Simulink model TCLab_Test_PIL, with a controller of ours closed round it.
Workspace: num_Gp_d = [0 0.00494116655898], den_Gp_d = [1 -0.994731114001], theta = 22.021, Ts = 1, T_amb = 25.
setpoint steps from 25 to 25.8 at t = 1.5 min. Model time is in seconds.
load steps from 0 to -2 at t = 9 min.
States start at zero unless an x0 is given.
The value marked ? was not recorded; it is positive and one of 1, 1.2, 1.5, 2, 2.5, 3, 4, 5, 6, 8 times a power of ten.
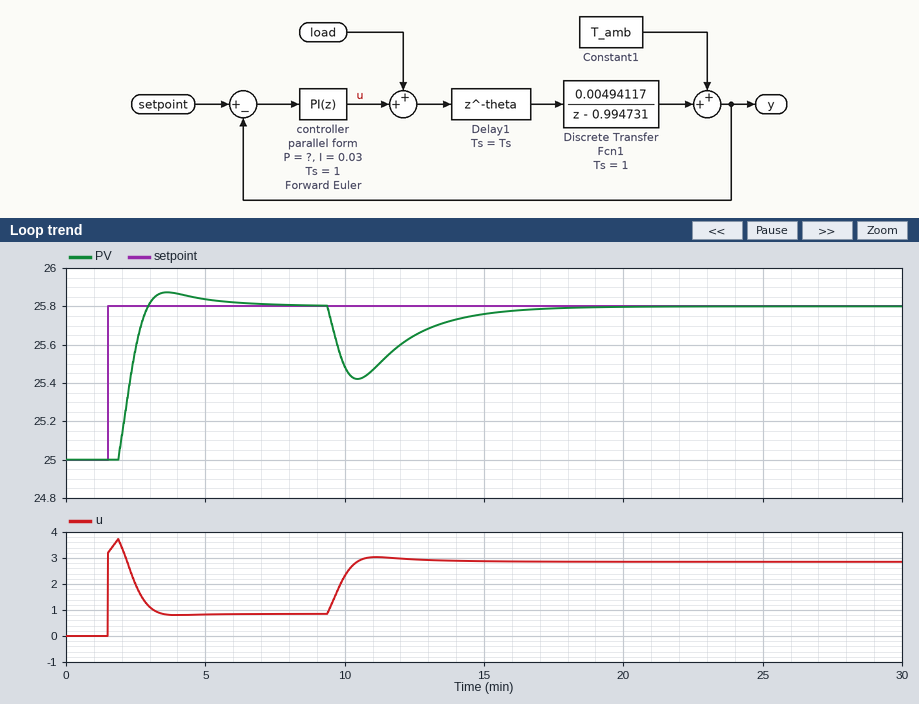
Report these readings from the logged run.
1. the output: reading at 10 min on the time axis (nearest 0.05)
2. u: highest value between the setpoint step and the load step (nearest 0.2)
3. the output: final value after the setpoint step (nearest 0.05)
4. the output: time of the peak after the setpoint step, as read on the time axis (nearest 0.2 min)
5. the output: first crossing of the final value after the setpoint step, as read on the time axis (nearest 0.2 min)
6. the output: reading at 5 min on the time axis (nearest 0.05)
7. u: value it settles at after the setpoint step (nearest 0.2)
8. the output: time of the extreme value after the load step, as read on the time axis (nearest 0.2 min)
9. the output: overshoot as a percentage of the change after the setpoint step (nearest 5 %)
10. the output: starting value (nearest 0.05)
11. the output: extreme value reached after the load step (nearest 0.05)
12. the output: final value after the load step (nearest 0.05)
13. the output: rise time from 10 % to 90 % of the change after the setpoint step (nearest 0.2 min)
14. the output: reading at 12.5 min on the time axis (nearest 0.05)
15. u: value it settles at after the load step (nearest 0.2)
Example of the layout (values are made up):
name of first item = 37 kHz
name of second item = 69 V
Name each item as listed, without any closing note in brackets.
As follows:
the output: reading at 10 min on the time axis = 25.50
u: highest value between the setpoint step and the load step = 3.8
the output: final value after the setpoint step = 25.80
the output: time of the peak after the setpoint step, as read on the time axis = 3.6 min
the output: first crossing of the final value after the setpoint step, as read on the time axis = 3.0 min
the output: reading at 5 min on the time axis = 25.85
u: value it settles at after the setpoint step = 0.8
the output: time of the extreme value after the load step, as read on the time axis = 10.4 min
the output: overshoot as a percentage of the change after the setpoint step = 10 %
the output: starting value = 25.00
the output: extreme value reached after the load step = 25.40
the output: final value after the load step = 25.80
the output: rise time from 10 % to 90 % of the change after the setpoint step = 0.8 min
the output: reading at 12.5 min on the time axis = 25.65
u: value it settles at after the load step = 2.8
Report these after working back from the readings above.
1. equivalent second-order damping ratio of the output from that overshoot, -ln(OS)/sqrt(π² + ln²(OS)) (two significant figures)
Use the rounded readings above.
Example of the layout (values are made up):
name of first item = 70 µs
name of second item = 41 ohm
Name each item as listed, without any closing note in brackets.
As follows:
equivalent second-order damping ratio of the output from that overshoot, -ln(OS)/sqrt(π² + ln²(OS)) = 0.59
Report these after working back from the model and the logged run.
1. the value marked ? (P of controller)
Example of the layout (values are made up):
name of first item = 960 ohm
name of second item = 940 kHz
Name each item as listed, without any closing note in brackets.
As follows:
the value marked ? = 4
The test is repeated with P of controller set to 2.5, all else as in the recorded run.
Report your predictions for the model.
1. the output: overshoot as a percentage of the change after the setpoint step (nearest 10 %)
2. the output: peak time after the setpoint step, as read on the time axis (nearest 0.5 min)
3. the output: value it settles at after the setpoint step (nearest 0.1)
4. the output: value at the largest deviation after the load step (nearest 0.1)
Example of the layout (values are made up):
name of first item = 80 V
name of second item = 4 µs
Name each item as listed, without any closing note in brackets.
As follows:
the output: overshoot as a percentage of the change after the setpoint step = 20 %
the output: peak time after the setpoint step, as read on the time axis = 4.5 min
the output: value it settles at after the setpoint step = 25.8
the output: value at the largest deviation after the load step = 25.3
